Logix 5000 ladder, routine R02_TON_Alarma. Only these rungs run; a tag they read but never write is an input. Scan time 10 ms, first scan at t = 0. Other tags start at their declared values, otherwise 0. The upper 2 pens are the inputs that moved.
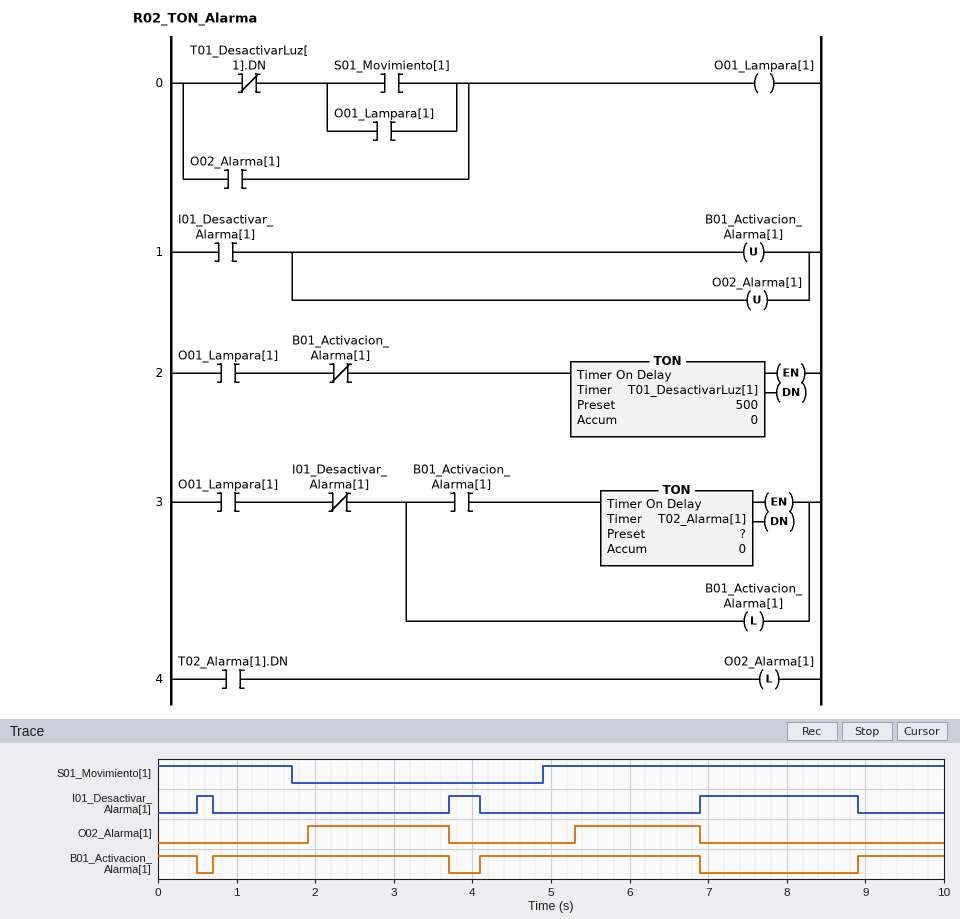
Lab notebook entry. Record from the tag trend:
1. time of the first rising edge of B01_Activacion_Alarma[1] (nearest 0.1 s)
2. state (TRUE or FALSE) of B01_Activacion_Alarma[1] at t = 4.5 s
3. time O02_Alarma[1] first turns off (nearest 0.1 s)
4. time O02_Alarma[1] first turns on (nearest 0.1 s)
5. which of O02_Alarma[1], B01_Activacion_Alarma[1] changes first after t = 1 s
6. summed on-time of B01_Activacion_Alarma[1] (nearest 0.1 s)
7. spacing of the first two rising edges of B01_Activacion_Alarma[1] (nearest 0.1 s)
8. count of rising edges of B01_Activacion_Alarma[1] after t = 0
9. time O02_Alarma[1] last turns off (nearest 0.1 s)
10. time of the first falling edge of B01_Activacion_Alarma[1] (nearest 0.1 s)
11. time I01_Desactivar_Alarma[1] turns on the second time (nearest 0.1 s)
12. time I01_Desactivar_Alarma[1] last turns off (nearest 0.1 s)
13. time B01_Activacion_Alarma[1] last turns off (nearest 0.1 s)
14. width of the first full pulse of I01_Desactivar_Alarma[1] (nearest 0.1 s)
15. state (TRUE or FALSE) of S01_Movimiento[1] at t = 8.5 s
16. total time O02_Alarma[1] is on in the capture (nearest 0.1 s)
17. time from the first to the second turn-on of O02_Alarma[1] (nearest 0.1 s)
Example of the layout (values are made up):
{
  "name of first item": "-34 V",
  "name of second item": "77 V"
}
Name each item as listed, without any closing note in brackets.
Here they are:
{
  "time of the first rising edge of B01_Activacion_Alarma[1]": "0.7 s",
  "state (TRUE or FALSE) of B01_Activacion_Alarma[1] at t = 4.5 s": "TRUE",
  "time O02_Alarma[1] first turns off": "3.7 s",
  "time O02_Alarma[1] first turns on": "1.9 s",
  "which of O02_Alarma[1], B01_Activacion_Alarma[1] changes first after t = 1 s": "O02_Alarma[1]",
  "summed on-time of B01_Activacion_Alarma[1]": "7.4 s",
  "spacing of the first two rising edges of B01_Activacion_Alarma[1]": "3.4 s",
  "count of rising edges of B01_Activacion_Alarma[1] after t = 0": "3",
  "time O02_Alarma[1] last turns off": "6.9 s",
  "time of the first falling edge of B01_Activacion_Alarma[1]": "0.5 s",
  "time I01_Desactivar_Alarma[1] turns on the second time": "3.7 s",
  "time I01_Desactivar_Alarma[1] last turns off": "8.9 s",
  "time B01_Activacion_Alarma[1] last turns off": "6.9 s",
  "width of the first full pulse of I01_Desactivar_Alarma[1]": "0.2 s",
  "state (TRUE or FALSE) of S01_Movimiento[1] at t = 8.5 s": "TRUE",
  "total time O02_Alarma[1] is on in the capture": "3.4 s",
  "time from the first to the second turn-on of O02_Alarma[1]": "3.4 s"
}
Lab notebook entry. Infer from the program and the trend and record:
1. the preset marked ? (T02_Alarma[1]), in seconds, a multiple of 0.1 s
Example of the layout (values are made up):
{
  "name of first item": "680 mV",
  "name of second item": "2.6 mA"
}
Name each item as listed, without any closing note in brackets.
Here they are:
{
  "the preset marked ? (T02_Alarma[1]), in seconds, a multiple of 0.1 s": "1.2 s"
}
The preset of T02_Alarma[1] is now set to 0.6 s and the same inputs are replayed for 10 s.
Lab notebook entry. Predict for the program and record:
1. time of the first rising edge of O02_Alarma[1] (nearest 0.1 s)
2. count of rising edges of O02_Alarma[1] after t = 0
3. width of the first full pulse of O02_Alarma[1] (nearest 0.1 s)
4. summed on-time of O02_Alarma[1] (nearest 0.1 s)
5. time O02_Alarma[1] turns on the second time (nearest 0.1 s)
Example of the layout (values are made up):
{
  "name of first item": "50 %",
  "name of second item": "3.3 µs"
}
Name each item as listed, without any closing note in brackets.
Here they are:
{
  "time of the first rising edge of O02_Alarma[1]": "1.3 s",
  "count of rising edges of O02_Alarma[1] after t = 0": "3",
  "width of the first full pulse of O02_Alarma[1]": "2.4 s",
  "summed on-time of O02_Alarma[1]": "5.1 s",
  "time O02_Alarma[1] turns on the second time": "4.7 s"
}
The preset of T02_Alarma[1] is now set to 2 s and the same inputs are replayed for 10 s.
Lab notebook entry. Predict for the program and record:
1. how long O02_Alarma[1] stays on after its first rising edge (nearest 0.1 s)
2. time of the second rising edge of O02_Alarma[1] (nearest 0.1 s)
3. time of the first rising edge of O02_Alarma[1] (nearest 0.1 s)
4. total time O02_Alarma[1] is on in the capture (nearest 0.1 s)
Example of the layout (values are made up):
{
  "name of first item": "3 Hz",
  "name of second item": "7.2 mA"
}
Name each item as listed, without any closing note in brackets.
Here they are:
{
  "how long O02_Alarma[1] stays on after its first rising edge": "1.0 s",
  "time of the second rising edge of O02_Alarma[1]": "6.1 s",
  "time of the first rising edge of O02_Alarma[1]": "2.7 s",
  "total time O02_Alarma[1] is on in the capture": "1.8 s"
}
